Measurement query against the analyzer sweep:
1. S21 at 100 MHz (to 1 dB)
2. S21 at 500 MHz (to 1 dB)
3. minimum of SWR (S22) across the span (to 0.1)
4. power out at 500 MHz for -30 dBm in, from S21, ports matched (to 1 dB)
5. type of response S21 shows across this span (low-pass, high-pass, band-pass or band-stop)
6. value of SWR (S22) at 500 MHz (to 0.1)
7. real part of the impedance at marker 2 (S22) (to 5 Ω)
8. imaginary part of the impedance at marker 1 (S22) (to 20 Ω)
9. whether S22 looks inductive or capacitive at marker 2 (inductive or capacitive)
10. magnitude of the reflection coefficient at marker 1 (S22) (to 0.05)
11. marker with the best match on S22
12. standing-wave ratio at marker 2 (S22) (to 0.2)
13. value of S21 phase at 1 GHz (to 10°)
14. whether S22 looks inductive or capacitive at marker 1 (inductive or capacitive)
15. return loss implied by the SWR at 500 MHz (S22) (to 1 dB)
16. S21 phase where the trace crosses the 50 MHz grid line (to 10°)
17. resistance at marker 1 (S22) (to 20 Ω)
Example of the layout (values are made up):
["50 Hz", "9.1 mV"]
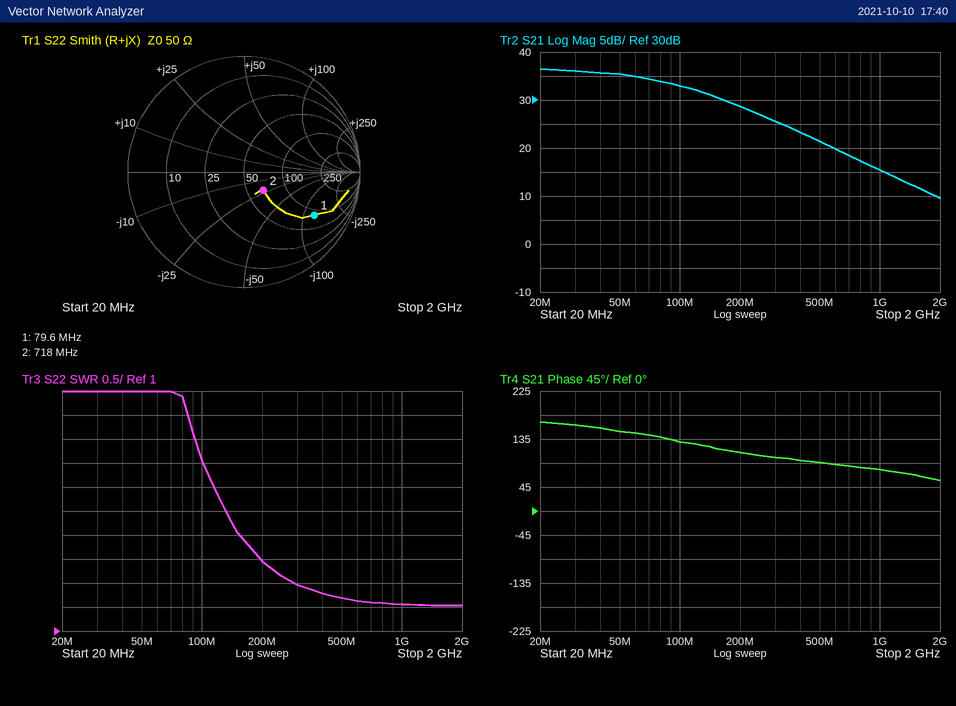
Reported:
["33 dB", "21 dB", "1.5", "-9 dBm", "low-pass", "1.7", "65 Ω", "-120 Ω", "capacitive", "0.70", "marker 2", "1.6", "80°", "capacitive", "12 dB", "150°", "80 Ω"]
